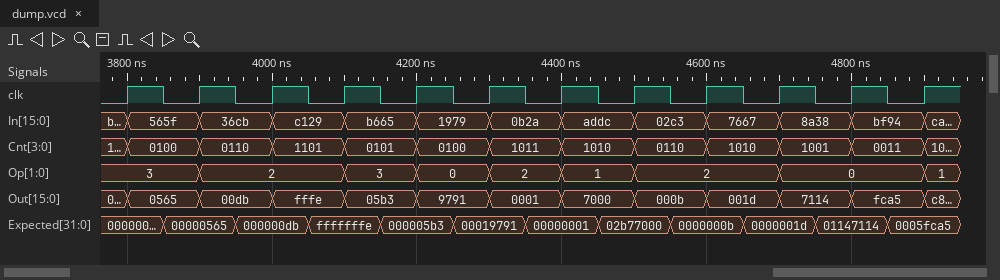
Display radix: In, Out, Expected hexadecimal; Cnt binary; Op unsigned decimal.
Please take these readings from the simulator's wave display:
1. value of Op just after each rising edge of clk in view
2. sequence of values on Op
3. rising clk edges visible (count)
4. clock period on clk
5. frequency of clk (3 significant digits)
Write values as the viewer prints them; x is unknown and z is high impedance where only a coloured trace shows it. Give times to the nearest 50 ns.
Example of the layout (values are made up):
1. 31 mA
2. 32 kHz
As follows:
1. 3, 2, 2, 3, 0, 2, 1, 2, 2, 0, 0, 1
2. 3, 2, 3, 0, 2, 1, 2, 0, 1
3. 12
4. 100 ns
5. 10.0 MHz
